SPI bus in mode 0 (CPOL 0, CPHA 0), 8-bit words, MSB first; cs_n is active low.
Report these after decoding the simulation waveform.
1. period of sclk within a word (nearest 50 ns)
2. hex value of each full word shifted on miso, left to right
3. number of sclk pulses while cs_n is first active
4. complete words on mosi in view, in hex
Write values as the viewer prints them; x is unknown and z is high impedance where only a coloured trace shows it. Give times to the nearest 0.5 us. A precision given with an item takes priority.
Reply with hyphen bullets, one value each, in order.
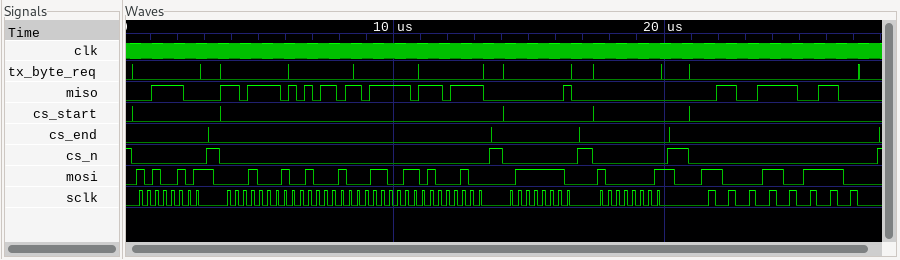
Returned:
- 300 ns
- 3C, DE, AD, BE, EF, 01, 00, 5A
- 8
- A5, 11, 22, 33, 44, 7E, 81, 96
